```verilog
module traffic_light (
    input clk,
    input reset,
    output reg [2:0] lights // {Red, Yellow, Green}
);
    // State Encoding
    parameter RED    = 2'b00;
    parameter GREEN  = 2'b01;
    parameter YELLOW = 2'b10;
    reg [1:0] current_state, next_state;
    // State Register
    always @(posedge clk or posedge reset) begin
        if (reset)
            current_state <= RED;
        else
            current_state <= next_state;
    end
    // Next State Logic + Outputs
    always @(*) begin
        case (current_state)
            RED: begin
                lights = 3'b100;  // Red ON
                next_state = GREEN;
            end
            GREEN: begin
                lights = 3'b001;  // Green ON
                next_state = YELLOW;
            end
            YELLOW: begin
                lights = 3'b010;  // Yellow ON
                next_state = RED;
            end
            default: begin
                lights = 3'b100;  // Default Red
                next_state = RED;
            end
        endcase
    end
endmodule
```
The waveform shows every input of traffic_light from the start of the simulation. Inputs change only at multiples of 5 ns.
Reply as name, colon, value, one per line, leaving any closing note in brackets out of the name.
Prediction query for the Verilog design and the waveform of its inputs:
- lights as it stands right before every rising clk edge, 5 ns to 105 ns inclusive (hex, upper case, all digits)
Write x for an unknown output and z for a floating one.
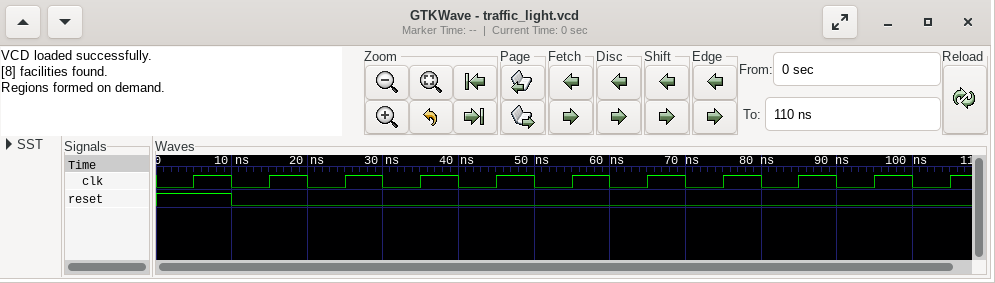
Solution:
lights as it stands right before every rising clk edge, 5 ns to 105 ns inclusive: 4, 4, 1, 2, 4, 1, 2, 4, 1, 2, 4
